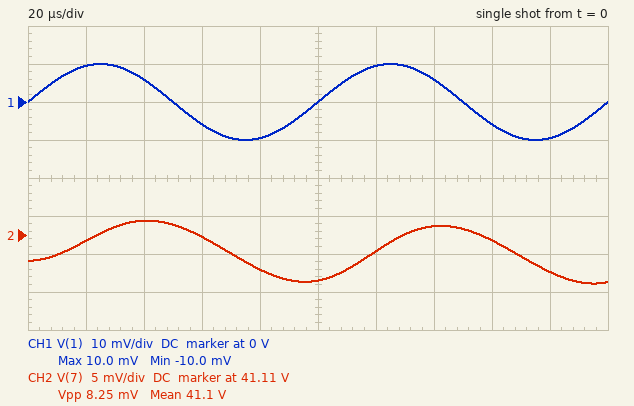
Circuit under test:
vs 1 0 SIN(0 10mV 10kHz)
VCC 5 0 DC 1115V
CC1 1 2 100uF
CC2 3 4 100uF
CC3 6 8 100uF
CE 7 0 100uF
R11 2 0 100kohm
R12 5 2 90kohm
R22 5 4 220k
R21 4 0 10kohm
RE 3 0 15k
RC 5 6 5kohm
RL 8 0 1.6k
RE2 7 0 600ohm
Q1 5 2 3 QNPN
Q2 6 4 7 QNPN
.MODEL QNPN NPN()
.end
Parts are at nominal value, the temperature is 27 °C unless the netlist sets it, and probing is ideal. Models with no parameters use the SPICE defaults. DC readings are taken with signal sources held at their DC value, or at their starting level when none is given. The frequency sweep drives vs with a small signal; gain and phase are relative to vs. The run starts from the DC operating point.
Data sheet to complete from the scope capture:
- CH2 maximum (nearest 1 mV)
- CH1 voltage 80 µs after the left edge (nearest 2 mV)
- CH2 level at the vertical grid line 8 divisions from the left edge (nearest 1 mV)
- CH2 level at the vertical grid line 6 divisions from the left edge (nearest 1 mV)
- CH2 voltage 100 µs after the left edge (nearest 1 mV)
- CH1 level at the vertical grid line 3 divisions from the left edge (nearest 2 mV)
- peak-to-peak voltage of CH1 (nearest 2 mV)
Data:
41.112 V
-10 mV
41.109 V
41.108 V
41.104 V
-6 mV
20 mV
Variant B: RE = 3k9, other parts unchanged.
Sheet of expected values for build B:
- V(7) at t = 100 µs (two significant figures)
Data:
41 V
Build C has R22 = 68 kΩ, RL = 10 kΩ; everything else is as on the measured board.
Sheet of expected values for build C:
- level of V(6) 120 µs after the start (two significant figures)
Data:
120 V
